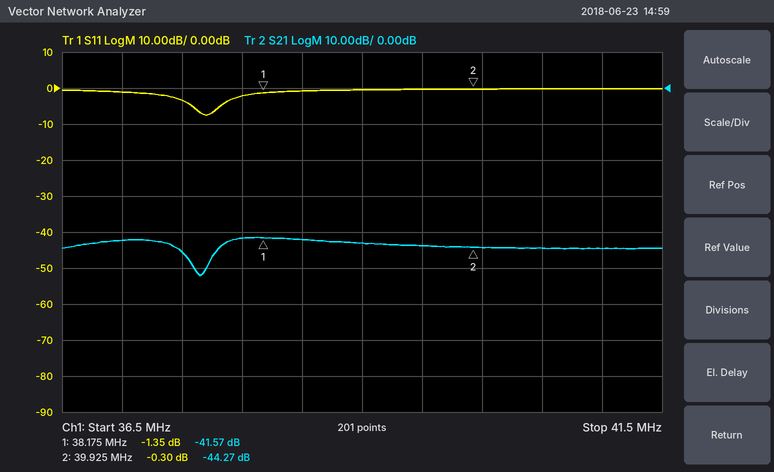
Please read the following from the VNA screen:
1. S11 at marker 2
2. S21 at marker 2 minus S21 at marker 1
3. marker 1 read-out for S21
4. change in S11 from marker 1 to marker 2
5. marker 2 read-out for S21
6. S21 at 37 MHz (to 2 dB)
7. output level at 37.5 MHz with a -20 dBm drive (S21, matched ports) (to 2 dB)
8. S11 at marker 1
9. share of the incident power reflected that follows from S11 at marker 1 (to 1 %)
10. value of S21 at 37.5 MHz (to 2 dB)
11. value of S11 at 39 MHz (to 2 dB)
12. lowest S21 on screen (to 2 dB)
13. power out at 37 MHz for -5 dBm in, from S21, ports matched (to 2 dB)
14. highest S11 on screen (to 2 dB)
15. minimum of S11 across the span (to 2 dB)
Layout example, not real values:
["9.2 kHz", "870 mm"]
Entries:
["-0.30 dB", "-2.70 dB", "-41.57 dB", "1.05 dB", "-44.27 dB", "-42 dB", "-66 dBm", "-1.35 dB", "73 %", "-46 dB", "0 dB", "-52 dB", "-48 dBm", "0 dB", "-8 dB"]
